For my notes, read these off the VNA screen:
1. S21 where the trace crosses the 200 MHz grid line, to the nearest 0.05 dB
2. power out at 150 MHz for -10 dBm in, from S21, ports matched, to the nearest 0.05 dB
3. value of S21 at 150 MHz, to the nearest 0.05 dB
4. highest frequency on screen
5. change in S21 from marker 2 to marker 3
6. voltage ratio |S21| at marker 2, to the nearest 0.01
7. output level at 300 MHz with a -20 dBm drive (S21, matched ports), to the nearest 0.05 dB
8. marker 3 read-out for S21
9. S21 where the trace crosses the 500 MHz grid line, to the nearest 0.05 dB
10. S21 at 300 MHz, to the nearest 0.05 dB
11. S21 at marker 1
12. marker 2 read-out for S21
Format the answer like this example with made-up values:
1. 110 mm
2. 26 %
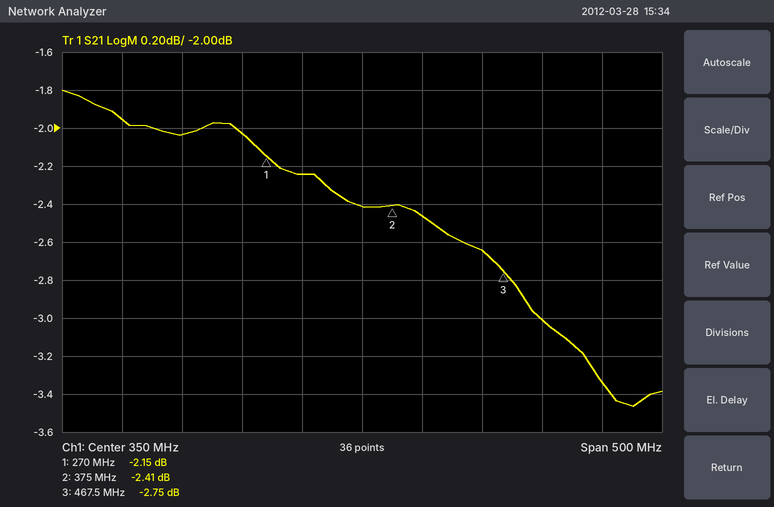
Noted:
1. -2.05 dB
2. -11.95 dBm
3. -1.95 dB
4. 600 MHz
5. -0.34 dB
6. 0.76
7. -22.25 dBm
8. -2.75 dB
9. -3.00 dB
10. -2.25 dB
11. -2.15 dB
12. -2.41 dB
